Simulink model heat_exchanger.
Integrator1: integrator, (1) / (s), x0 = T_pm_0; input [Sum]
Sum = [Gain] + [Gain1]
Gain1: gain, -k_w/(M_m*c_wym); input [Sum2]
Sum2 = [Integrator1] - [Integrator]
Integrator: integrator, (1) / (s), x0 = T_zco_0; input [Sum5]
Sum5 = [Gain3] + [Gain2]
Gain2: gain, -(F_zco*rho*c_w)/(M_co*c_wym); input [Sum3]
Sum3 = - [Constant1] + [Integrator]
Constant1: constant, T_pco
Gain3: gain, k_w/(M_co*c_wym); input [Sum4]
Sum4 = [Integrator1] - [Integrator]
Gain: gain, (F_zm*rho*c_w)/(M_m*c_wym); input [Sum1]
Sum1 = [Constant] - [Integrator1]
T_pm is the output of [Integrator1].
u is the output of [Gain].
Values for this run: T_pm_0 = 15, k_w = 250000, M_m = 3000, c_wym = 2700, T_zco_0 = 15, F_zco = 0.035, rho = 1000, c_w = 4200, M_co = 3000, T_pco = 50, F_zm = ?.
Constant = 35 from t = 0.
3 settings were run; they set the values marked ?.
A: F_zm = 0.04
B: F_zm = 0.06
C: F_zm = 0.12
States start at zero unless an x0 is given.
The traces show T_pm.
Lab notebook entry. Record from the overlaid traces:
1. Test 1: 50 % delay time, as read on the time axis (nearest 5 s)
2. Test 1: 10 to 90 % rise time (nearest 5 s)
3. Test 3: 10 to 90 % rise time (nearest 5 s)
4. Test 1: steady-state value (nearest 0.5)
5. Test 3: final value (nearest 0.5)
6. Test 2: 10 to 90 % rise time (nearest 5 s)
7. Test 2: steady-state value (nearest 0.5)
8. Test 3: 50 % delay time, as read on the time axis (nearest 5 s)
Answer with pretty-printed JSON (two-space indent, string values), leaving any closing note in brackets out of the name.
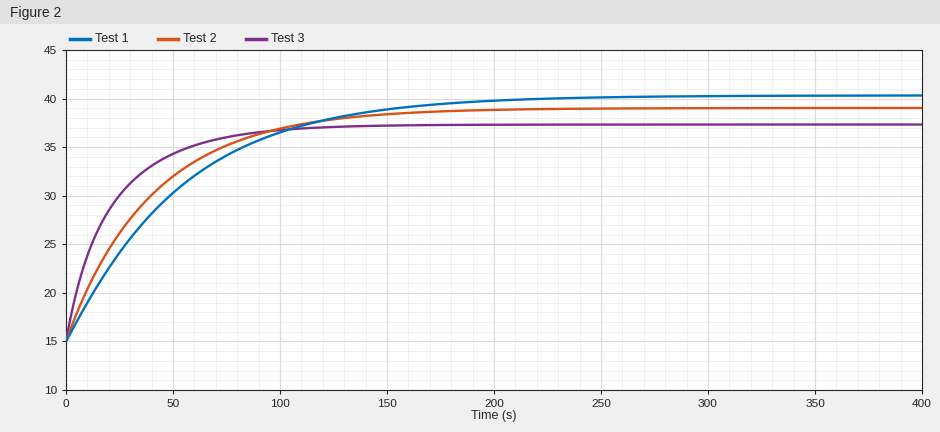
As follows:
{
  "Test 1: 50 % delay time, as read on the time axis": "40 s",
  "Test 1: 10 to 90 % rise time": "115 s",
  "Test 3: 10 to 90 % rise time": "55 s",
  "Test 1: steady-state value": "40.5",
  "Test 3: final value": "37.5",
  "Test 2: 10 to 90 % rise time": "90 s",
  "Test 2: steady-state value": "39.0",
  "Test 3: 50 % delay time, as read on the time axis": "15 s"
}
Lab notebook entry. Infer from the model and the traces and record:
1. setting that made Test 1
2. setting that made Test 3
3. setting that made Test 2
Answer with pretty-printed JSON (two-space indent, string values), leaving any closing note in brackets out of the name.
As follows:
{
  "setting that made Test 1": "A",
  "setting that made Test 3": "C",
  "setting that made Test 2": "B"
}
